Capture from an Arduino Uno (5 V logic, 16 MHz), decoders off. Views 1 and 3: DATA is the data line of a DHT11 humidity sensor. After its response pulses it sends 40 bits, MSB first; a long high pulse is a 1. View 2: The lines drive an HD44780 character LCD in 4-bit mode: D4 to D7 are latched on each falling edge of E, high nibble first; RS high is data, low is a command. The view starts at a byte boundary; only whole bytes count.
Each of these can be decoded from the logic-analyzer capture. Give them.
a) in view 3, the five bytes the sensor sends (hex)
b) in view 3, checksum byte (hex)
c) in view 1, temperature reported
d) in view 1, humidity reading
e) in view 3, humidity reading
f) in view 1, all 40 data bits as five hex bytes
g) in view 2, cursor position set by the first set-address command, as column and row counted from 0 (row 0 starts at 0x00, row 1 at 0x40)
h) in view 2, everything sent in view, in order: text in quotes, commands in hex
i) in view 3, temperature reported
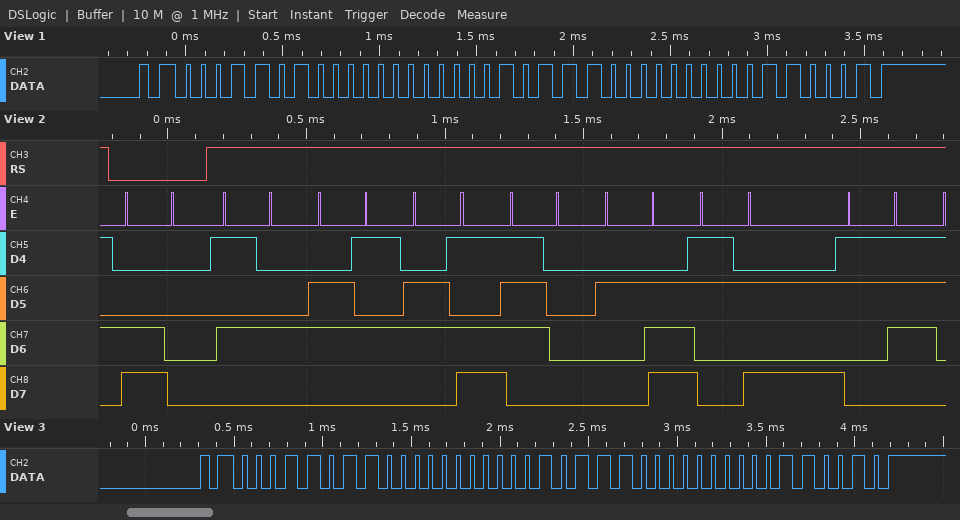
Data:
1B 00 17 00 32
0x32
23.0 °C
26 %
27 %
1A 00 17 00 31
column 0, row 1
0xC0 "Temp.:7"
23.0 °C
